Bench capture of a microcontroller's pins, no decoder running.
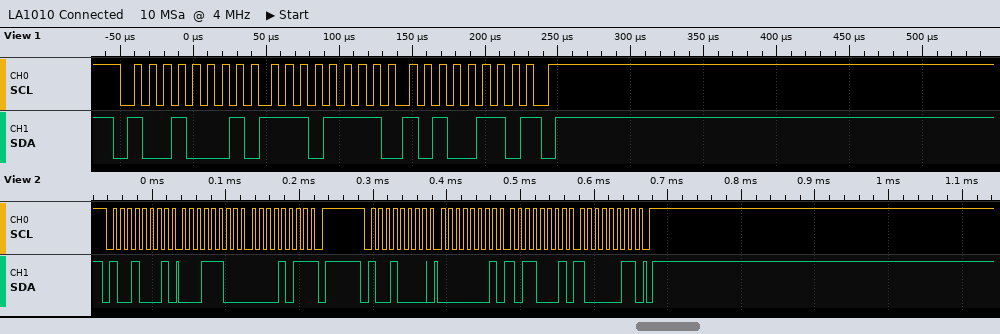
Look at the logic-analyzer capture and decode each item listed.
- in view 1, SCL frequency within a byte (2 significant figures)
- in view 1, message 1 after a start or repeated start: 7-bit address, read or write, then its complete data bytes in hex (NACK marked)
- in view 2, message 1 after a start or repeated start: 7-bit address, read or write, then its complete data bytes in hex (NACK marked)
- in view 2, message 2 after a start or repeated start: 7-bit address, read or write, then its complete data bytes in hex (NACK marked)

100 kHz
0x48 read: EF A6 NACK
0x48 read: 1C 0B NACK
0x48 write: 01 B1 83
